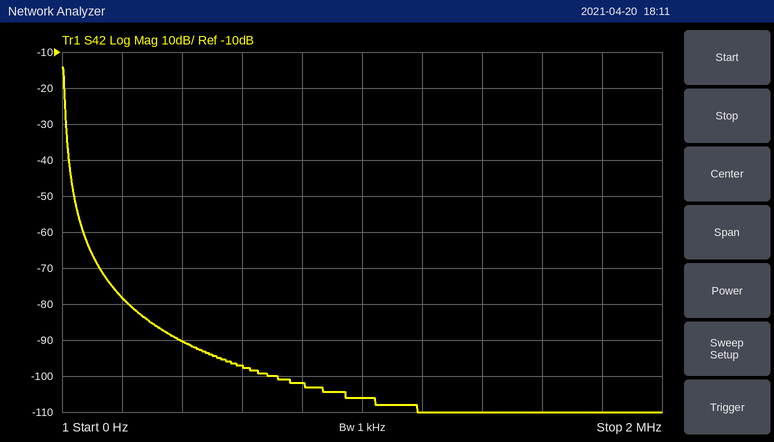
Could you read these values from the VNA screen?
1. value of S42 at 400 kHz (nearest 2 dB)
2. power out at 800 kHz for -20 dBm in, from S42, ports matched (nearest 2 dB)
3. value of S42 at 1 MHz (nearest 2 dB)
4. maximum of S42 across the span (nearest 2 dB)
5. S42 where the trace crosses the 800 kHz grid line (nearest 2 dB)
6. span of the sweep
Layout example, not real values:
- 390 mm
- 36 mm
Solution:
- -90 dB
- -122 dBm
- -106 dB
- -14 dB
- -102 dB
- 2 MHz
